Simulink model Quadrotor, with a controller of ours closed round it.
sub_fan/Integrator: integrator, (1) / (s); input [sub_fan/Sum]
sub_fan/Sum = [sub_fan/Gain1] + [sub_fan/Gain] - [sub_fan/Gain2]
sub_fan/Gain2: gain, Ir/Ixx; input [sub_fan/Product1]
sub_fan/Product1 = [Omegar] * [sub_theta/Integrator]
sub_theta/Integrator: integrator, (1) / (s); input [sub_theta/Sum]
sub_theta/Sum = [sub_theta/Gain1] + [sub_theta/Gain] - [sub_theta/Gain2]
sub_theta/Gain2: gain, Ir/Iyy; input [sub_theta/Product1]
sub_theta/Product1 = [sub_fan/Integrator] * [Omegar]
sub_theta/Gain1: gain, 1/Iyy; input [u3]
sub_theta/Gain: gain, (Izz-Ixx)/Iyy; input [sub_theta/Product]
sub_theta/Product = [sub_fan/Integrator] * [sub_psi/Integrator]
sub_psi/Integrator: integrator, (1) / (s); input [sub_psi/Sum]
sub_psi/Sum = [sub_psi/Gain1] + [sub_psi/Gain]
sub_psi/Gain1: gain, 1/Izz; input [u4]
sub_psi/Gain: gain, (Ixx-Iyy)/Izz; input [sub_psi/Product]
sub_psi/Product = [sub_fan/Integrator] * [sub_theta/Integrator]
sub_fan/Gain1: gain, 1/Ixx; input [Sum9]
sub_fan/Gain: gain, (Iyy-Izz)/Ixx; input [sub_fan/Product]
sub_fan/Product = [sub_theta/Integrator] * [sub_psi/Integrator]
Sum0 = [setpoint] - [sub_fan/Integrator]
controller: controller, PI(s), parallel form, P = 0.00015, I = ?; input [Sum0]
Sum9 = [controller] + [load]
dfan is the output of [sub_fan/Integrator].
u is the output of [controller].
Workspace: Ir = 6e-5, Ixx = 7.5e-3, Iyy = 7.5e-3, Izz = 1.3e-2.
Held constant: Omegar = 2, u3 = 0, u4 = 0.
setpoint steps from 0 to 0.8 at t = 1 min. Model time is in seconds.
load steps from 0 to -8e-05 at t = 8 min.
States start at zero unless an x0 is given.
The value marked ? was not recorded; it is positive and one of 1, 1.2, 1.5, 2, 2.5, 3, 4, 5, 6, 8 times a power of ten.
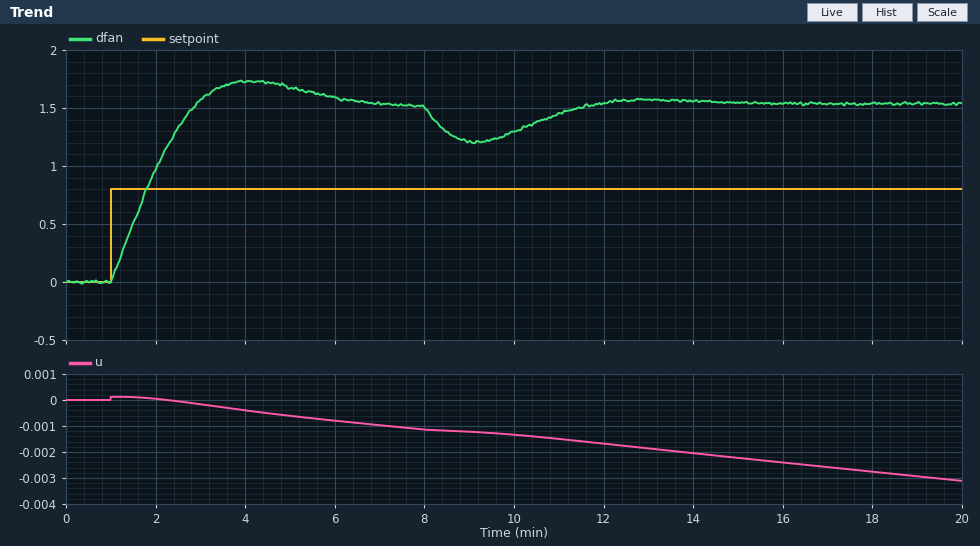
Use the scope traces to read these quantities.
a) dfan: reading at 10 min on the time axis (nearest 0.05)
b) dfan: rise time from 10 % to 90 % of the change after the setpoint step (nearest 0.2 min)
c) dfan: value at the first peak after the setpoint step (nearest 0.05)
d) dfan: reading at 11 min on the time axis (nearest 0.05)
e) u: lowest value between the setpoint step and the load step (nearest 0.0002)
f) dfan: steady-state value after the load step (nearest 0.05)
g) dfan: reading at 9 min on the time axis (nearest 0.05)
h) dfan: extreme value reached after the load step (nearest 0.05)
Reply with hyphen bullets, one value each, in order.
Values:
- 1.30
- 1.4 min
- 1.75
- 1.45
- -0.0012
- 1.55
- 1.20
- 1.20
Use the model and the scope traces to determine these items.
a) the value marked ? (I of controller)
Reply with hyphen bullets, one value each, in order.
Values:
- 4e-06
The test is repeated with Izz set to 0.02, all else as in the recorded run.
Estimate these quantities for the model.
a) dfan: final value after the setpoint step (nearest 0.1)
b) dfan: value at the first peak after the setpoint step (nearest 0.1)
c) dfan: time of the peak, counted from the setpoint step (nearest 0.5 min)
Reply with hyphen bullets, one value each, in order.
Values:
- 1.5
- 1.7
- 3.0 min
